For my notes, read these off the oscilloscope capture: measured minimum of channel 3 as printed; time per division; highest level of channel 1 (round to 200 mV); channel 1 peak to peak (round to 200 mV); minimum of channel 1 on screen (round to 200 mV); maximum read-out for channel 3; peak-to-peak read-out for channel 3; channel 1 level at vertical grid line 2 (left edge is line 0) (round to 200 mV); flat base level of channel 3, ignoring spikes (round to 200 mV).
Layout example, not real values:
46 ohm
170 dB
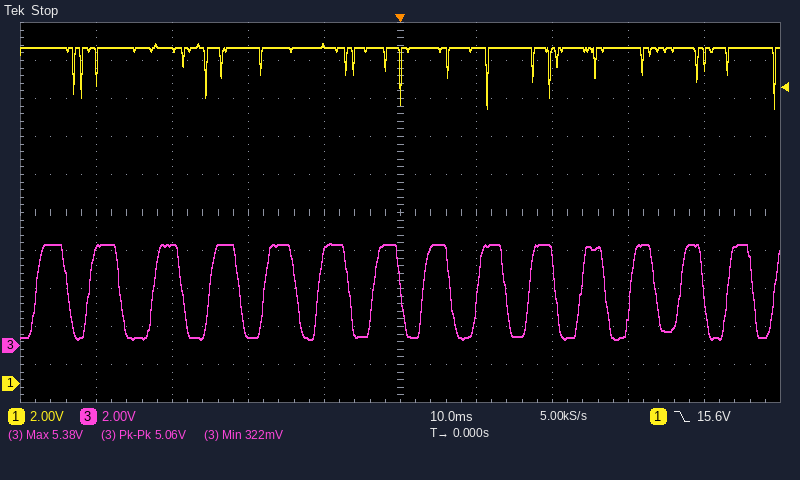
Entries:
322 mV
10 ms
17.8 V
3.4 V
14.4 V
5.38 V
5.06 V
17.6 V
400 mV
